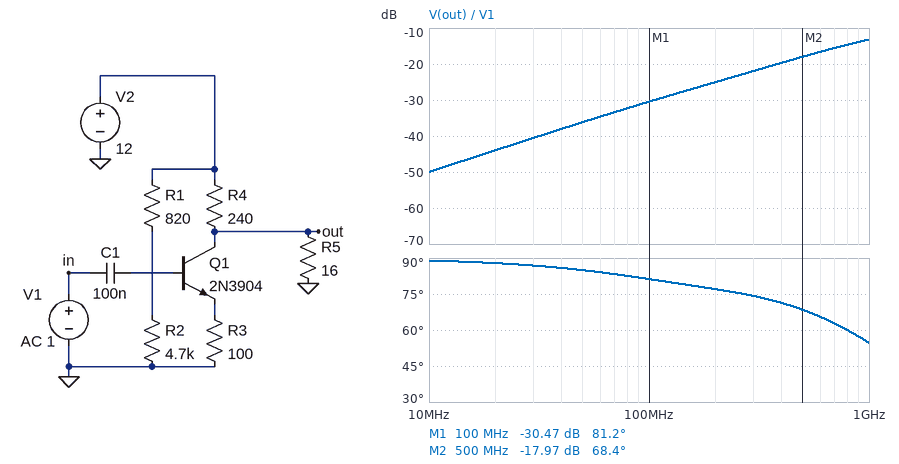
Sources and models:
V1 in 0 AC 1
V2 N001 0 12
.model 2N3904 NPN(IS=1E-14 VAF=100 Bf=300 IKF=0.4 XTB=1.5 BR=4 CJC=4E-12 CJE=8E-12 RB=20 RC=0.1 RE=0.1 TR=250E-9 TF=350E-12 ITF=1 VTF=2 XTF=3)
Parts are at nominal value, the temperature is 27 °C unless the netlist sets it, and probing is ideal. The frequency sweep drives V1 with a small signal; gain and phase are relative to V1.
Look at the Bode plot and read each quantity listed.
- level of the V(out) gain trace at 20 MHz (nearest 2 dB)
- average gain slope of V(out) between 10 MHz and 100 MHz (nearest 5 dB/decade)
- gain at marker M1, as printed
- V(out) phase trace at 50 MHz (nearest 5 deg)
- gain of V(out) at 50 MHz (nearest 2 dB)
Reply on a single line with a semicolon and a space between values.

-44 dB; 20 dB/decade; -30.47 dB; 85 deg; -36 dB
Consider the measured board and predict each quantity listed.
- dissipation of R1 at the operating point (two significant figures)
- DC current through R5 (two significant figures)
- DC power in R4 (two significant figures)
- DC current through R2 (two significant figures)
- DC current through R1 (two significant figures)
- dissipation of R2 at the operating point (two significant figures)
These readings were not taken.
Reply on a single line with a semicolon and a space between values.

3.9 mW; 47 mA; 530 mW; 2.2 mA; 2.2 mA; 22 mW
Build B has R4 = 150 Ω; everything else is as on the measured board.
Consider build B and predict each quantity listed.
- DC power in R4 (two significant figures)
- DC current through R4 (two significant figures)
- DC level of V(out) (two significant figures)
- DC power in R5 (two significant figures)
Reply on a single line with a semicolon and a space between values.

780 mW; 72 mA; 1.2 V; 84 mW
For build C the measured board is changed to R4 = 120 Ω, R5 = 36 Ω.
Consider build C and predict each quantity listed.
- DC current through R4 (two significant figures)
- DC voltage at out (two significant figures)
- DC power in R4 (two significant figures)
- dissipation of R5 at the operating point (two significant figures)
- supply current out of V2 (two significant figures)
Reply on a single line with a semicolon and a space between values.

77 mA; 2.8 V; 710 mW; 210 mW; 79 mA
